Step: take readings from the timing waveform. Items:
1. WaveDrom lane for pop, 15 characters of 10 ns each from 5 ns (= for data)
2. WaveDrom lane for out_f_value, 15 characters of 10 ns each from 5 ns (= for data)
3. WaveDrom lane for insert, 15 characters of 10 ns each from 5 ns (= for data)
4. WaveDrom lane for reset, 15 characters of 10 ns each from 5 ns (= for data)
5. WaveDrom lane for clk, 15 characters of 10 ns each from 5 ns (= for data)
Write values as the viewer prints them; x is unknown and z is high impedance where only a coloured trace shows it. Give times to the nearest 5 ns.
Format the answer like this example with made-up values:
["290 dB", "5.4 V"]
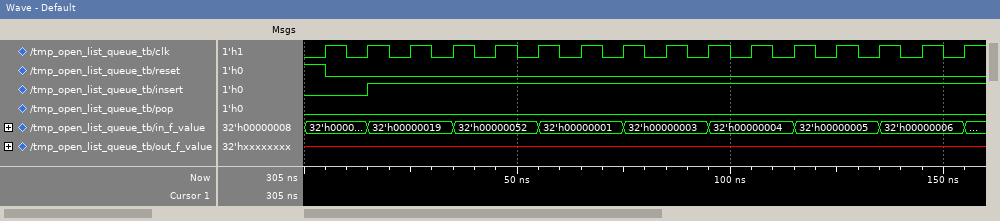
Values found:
["{name: 'pop', wave: '0..............'}", "{name: 'out_f_value', wave: 'x..............'}", "{name: 'insert', wave: '01.............'}", "{name: 'reset', wave: '0..............'}", "{name: 'clk', wave: 'p..............'}"]
